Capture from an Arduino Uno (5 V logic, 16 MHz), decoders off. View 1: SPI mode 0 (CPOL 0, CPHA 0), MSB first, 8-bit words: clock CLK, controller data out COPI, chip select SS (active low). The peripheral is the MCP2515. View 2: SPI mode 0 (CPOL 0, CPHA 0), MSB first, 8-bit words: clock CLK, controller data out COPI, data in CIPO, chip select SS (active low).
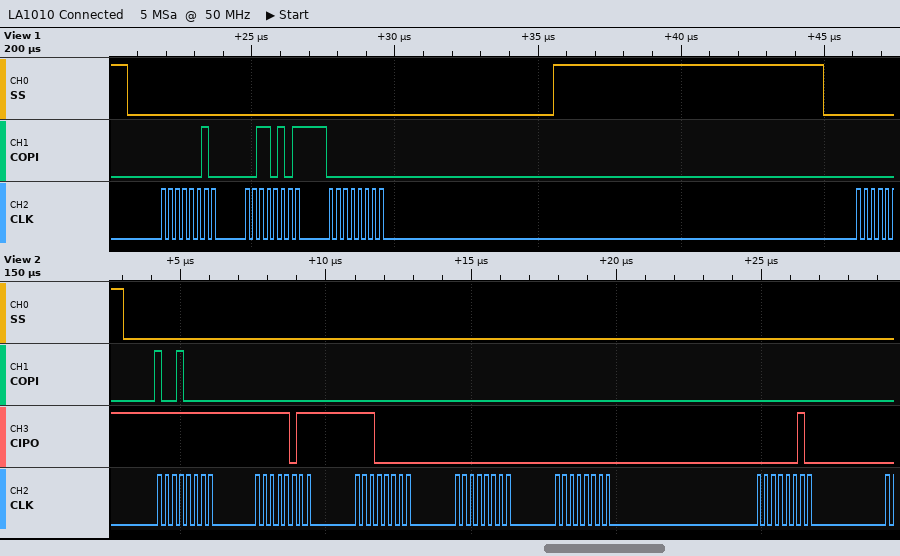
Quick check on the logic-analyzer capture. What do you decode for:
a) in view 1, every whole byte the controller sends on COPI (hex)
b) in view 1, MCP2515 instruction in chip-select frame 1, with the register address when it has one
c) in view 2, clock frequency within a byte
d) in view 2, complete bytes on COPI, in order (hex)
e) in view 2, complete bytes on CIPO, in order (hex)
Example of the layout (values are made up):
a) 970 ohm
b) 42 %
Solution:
a) 02 35 00
b) WRITE 0x35
c) 4 MHz
d) 90 00 00 00 00 00
e) FF FB E0 00 00 02
